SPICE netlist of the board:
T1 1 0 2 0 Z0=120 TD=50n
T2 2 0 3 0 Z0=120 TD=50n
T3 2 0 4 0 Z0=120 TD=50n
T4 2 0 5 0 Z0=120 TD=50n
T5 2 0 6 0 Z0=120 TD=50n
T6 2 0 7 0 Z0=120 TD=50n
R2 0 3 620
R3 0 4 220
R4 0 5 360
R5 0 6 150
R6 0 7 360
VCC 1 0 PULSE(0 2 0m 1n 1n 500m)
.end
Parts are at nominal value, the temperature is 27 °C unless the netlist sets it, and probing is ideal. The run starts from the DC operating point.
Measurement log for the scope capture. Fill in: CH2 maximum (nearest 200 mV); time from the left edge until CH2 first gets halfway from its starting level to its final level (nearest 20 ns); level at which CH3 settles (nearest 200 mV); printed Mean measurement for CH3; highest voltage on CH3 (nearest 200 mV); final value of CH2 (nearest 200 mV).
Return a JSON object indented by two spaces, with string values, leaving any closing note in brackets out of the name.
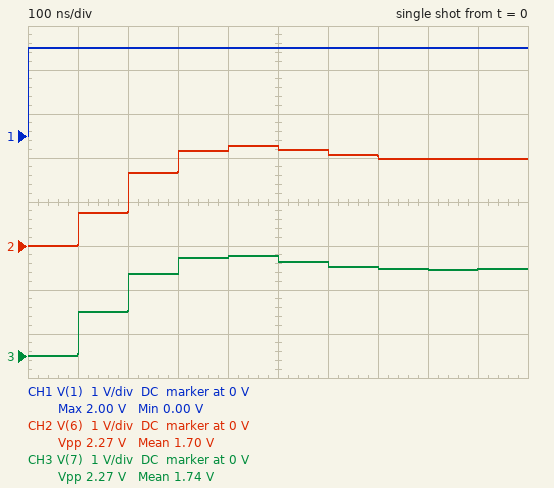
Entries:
{
  "CH2 maximum": "2.2 V",
  "time from the left edge until CH2 first gets halfway from its starting level to its final level": "200 ns",
  "level at which CH3 settles": "2.0 V",
  "printed Mean measurement for CH3": "1.74 V",
  "highest voltage on CH3": "2.2 V",
  "final value of CH2": "2.0 V"
}
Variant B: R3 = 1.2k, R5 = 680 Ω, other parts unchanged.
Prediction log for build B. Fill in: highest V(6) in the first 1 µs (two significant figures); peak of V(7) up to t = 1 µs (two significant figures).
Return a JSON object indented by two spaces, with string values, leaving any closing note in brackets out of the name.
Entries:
{
  "highest V(6) in the first 1 µs": "2.9 V",
  "peak of V(7) up to t = 1 µs": "2.8 V"
}
